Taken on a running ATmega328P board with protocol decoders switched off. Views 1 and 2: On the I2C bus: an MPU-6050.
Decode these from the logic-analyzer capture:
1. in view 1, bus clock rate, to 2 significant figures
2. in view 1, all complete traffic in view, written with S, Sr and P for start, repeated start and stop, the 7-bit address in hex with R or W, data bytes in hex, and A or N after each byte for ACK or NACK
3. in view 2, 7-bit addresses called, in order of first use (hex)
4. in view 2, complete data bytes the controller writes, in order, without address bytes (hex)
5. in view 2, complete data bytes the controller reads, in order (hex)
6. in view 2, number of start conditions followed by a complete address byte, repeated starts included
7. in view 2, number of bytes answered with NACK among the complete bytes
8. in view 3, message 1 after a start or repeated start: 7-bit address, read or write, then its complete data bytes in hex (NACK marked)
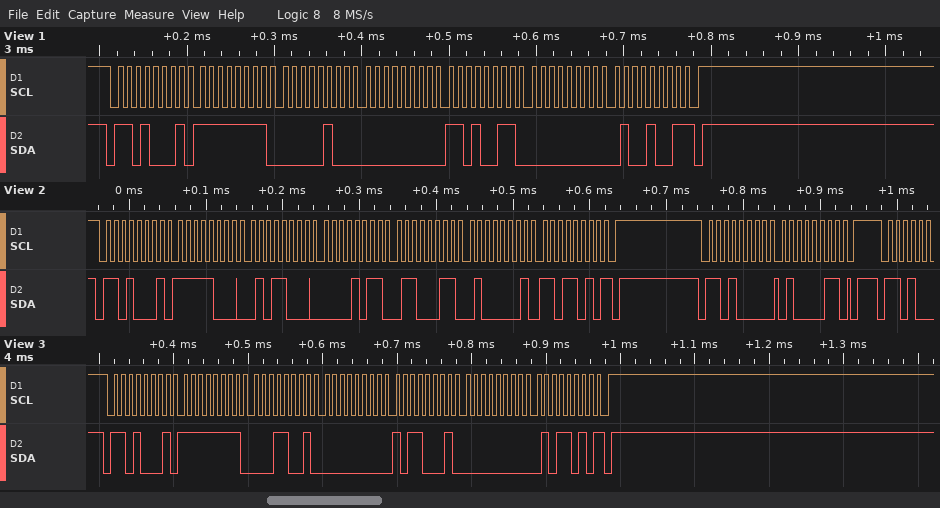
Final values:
100 kHz
S 68R A FF A 04 A 00 A D3 A 00 A 49 N P
0x68
43
F8 58 0B 63 41 DA
2
1
0x68 read: FF 19 00 B1 00 5A NACK
